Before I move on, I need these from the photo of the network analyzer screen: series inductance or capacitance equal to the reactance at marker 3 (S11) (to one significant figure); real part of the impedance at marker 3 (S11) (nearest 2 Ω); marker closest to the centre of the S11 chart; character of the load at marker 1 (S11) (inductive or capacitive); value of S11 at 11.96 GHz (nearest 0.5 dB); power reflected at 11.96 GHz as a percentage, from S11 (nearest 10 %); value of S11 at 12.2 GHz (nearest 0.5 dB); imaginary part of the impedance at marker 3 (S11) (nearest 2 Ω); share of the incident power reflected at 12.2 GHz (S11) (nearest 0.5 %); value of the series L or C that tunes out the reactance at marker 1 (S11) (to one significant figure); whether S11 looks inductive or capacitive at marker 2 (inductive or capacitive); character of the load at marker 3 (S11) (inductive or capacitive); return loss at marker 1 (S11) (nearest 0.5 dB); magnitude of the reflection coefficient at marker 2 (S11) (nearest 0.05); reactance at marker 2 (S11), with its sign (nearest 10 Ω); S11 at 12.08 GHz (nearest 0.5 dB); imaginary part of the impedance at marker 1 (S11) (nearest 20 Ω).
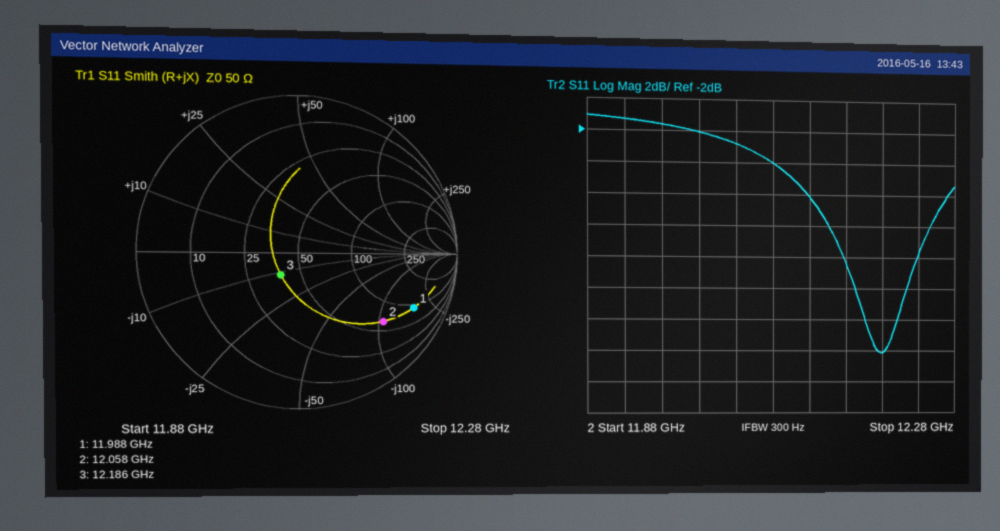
1 pF
38 Ω
marker 3
capacitive
-1.5 dB
70 %
-16.0 dB
-12 Ω
2.5 %
2 nH
capacitive
capacitive
2.0 dB
0.70
-110 Ω
-4.0 dB
-180 Ω
